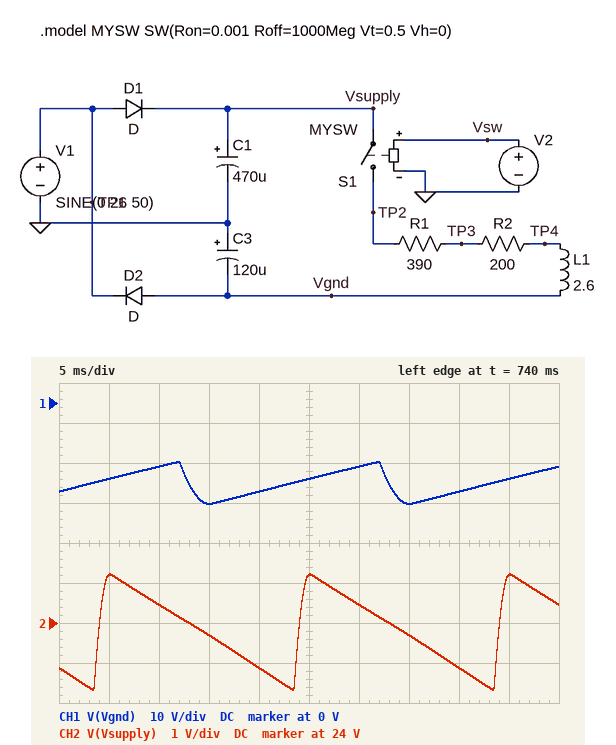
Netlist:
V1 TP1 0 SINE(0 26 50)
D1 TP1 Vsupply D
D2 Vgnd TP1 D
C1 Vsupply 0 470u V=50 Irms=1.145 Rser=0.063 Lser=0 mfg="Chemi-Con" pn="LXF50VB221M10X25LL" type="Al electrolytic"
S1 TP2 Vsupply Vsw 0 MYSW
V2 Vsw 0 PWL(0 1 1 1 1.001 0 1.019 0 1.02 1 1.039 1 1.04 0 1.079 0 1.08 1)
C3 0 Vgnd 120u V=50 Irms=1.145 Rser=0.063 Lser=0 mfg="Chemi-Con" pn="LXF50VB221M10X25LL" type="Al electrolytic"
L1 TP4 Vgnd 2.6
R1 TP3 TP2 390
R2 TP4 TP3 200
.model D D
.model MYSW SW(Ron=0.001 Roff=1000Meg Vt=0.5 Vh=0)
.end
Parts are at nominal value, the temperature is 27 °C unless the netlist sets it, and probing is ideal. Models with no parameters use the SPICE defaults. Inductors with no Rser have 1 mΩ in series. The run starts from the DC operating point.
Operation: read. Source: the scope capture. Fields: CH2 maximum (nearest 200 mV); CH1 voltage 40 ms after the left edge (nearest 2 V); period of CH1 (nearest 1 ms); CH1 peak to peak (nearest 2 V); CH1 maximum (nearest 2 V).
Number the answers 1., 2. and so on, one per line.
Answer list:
1. 25.2 V
2. -22 V
3. 20 ms
4. 10 V
5. -14 V
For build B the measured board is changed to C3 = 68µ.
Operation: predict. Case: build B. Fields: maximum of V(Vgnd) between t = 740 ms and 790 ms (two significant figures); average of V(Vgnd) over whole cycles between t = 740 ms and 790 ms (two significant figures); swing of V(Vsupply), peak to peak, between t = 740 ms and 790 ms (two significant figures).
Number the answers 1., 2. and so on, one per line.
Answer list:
1. -8.6 V
2. -17 V
3. 2.7 V
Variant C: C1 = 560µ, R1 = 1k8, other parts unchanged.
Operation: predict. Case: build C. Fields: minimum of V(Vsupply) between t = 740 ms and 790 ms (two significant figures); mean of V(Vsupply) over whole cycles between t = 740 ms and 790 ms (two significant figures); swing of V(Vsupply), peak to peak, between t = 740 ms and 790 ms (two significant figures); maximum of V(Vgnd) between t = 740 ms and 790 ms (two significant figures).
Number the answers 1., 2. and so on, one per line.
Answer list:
1. 24 V
2. 25 V
3. 820 mV
4. -22 V
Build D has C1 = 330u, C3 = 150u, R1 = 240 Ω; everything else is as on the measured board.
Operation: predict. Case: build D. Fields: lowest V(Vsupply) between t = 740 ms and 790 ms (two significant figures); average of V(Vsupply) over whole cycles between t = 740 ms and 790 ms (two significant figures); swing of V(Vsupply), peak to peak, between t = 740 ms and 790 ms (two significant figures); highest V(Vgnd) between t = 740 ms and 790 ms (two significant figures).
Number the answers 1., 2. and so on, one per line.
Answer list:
1. 20 V
2. 23 V
3. 5.2 V
4. -14 V
